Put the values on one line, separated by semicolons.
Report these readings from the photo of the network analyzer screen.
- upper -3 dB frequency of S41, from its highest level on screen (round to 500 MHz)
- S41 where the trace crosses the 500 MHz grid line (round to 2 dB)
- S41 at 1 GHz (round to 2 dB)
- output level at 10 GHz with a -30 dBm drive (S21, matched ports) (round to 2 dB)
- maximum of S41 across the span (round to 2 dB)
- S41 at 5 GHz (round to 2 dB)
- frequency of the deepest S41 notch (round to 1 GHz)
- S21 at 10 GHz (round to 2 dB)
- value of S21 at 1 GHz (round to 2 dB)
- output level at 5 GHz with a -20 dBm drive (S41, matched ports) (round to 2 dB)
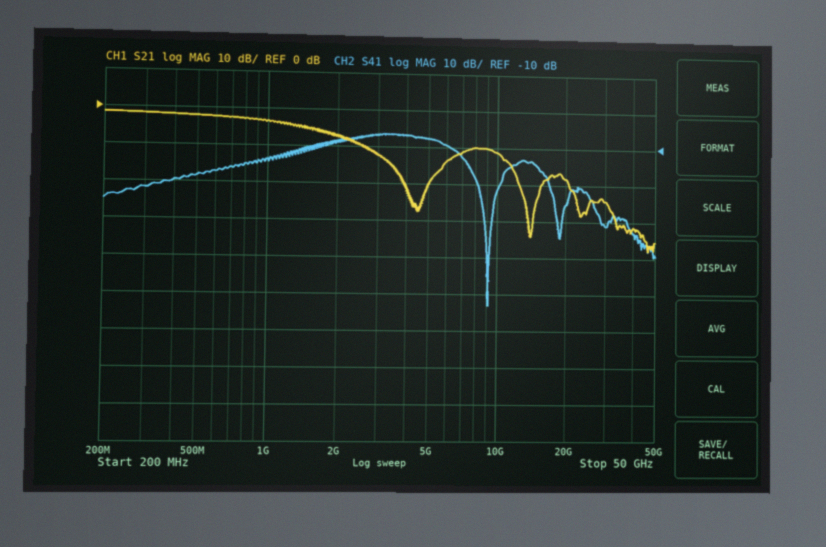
6.0 GHz; -18 dB; -14 dB; -42 dBm; -6 dB; -8 dB; 9 GHz; -12 dB; -4 dB; -28 dBm
